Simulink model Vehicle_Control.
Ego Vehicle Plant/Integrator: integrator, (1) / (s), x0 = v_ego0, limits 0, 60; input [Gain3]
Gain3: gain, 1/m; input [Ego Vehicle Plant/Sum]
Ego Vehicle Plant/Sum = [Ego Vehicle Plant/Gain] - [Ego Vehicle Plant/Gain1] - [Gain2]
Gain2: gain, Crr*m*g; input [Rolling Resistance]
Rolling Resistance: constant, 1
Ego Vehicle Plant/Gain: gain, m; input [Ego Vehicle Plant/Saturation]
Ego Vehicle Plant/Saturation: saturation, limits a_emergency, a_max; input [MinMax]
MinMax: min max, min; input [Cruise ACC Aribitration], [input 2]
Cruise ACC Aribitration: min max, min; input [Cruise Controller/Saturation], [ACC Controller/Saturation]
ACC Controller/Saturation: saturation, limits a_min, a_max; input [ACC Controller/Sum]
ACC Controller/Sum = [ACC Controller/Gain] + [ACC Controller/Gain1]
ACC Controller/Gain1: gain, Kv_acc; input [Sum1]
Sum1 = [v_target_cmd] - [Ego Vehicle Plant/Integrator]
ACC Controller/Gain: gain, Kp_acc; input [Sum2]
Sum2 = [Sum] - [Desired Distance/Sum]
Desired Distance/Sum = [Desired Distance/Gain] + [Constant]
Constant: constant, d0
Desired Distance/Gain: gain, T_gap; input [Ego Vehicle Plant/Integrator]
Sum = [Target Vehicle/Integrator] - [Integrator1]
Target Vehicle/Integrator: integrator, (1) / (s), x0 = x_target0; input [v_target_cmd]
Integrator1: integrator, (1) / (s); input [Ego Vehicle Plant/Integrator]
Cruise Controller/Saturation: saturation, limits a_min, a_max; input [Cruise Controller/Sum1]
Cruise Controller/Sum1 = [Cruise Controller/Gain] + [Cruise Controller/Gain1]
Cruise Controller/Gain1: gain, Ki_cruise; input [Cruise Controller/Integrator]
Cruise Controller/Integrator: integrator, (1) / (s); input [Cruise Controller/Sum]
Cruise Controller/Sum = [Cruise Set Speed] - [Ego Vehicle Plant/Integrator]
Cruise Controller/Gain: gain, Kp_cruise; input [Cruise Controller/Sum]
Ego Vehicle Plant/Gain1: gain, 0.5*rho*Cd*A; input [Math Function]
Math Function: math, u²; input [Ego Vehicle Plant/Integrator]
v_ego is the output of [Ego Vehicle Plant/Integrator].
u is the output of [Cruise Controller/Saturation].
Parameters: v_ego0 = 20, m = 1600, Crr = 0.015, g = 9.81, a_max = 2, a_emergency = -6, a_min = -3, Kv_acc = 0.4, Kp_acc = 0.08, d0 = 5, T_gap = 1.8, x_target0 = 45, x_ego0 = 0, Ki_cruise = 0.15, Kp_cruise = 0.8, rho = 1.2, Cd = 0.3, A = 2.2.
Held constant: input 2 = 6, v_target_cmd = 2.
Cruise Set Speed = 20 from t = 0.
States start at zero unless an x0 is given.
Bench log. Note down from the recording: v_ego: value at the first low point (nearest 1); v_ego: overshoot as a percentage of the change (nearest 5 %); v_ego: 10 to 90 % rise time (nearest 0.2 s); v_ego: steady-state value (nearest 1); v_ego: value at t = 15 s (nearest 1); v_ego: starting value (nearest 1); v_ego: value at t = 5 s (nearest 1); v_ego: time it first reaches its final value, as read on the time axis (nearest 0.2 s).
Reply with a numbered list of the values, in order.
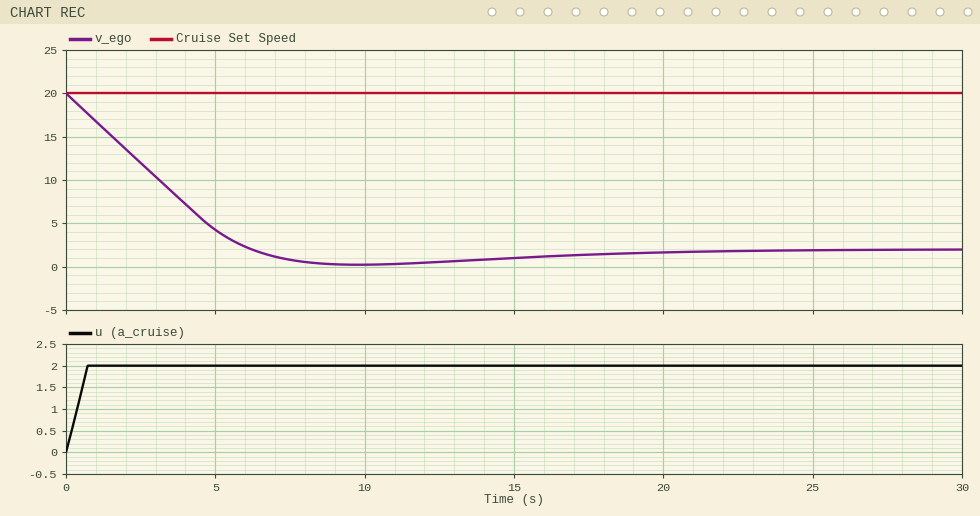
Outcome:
1. 0
2. 10 %
3. 4.6 s
4. 2
5. 1
6. 20
7. 4
8. 6.2 s
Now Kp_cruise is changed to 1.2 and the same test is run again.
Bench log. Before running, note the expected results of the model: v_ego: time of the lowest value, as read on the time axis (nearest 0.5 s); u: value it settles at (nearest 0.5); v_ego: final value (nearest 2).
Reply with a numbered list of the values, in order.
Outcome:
1. 10.0 s
2. 2.0
3. 2
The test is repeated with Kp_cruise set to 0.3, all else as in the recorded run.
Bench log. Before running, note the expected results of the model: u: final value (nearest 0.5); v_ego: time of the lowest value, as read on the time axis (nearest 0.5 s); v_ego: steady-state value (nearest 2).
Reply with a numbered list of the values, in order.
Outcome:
1. 2.0
2. 10.0 s
3. 2
